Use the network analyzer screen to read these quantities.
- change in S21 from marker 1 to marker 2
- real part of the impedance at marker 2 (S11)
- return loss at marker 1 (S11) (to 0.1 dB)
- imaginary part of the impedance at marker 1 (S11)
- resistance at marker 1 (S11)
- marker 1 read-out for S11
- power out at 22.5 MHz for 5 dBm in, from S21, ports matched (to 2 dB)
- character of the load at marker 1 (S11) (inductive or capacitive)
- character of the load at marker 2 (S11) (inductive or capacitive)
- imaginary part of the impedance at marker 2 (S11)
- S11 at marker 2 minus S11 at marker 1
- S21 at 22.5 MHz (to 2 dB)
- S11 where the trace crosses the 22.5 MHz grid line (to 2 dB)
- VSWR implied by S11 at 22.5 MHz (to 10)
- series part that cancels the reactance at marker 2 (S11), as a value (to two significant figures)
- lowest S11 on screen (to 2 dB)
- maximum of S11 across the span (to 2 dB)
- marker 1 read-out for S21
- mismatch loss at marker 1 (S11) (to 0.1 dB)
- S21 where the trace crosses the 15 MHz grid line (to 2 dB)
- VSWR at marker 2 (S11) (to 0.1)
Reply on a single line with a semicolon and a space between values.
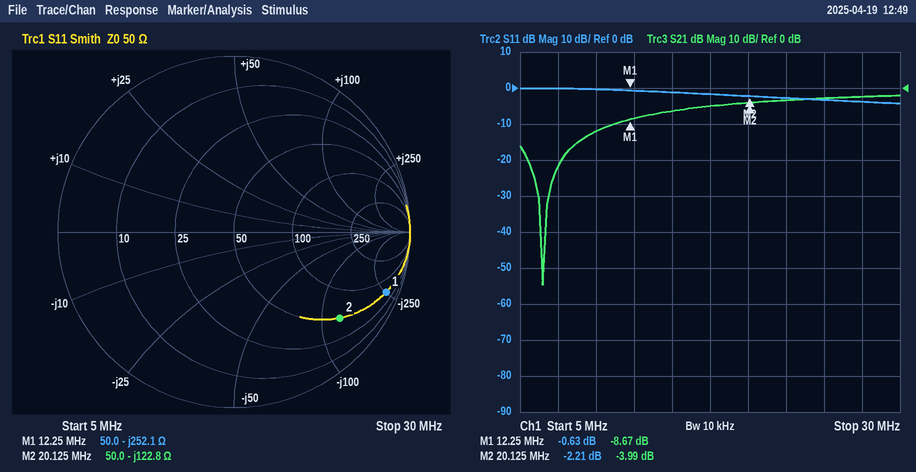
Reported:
4.68 dB; 50.0 Ω; 0.6 dB; -252.1 Ω; 50.0 Ω; -0.63 dB; 2 dBm; capacitive; capacitive; -122.8 Ω; -1.58 dB; -4 dB; -2 dB; 10; 970 nH; -4 dB; 0 dB; -8.67 dB; 8.7 dB; -6 dB; 7.9
